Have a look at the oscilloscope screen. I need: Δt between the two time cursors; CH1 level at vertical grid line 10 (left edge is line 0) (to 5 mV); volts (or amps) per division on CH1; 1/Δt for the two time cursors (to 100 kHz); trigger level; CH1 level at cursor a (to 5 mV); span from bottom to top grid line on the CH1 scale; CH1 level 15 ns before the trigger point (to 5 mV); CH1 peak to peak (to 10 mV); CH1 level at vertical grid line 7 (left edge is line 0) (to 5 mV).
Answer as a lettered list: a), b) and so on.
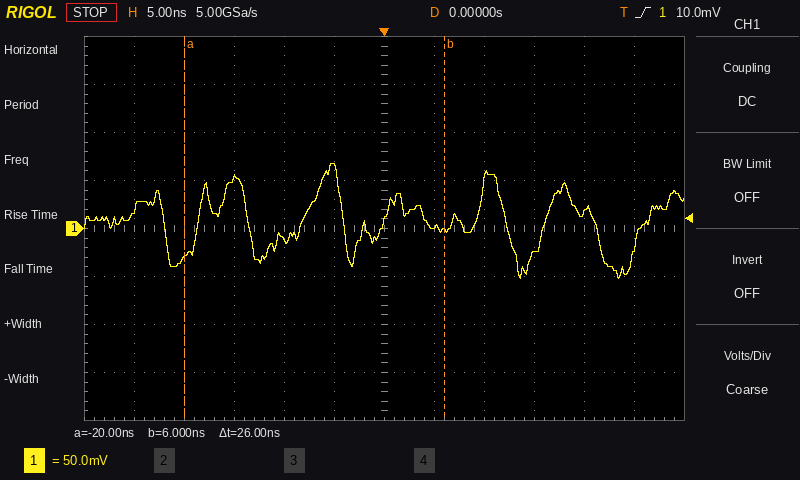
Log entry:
a) 26 ns
b) 15 mV
c) 50 mV
d) 38.5 MHz
e) 10.0 mV
f) -30 mV
g) 400 mV
h) 50 mV
i) 120 mV
j) 0 mV
